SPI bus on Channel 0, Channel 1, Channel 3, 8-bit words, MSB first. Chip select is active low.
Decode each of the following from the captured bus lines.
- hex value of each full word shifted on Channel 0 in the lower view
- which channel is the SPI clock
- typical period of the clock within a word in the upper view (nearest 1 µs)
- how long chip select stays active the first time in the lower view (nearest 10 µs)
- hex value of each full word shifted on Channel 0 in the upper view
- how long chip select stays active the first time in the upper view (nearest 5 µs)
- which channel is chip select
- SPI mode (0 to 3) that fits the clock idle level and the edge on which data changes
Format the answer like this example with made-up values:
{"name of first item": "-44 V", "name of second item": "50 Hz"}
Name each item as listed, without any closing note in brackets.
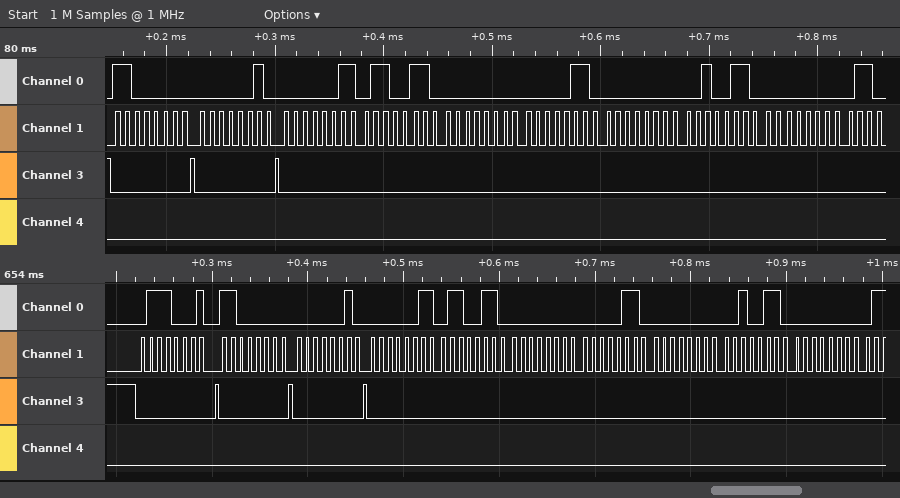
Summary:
{"hex value of each full word shifted on Channel 0 in the lower view": "71, C0, 02, 03, 66, 00, 06, 00, 26, 00", "which channel is the SPI clock": "Channel 1", "typical period of the clock within a word in the upper view": "9 µs", "how long chip select stays active the first time in the lower view": "80 µs", "hex value of each full word shifted on Channel 0 in the upper view": "C0, 02, 03, 66, 00, 06, 00, 26, 00", "how long chip select stays active the first time in the upper view": "75 µs", "which channel is chip select": "Channel 3", "SPI mode (0 to 3) that fits the clock idle level and the edge on which data changes": "0"}
